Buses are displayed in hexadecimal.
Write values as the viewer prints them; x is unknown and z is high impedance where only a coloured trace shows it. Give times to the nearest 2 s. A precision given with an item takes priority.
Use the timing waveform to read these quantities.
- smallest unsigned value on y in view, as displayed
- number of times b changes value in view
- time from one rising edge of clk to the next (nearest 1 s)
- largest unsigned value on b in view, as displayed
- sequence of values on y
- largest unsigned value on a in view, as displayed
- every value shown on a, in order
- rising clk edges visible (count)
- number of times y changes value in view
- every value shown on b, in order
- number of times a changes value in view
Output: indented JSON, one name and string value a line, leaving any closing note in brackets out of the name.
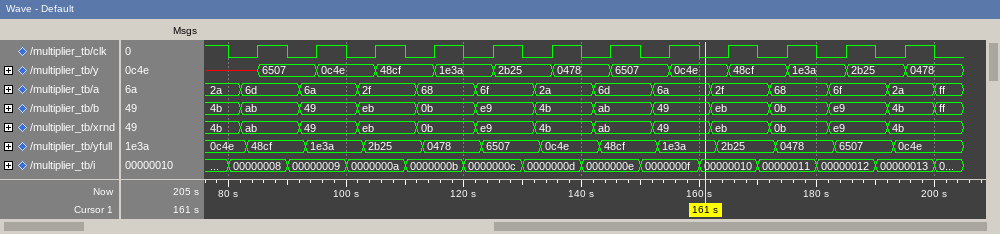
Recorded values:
{
  "smallest unsigned value on y in view, as displayed": "0478",
  "number of times b changes value in view": "13",
  "time from one rising edge of clk to the next": "10 s",
  "largest unsigned value on b in view, as displayed": "ff",
  "sequence of values on y": "x, 6507, 0c4e, 48cf, 1e3a, 2b25, 0478, 6507, 0c4e, 48cf, 1e3a, 2b25, 0478",
  "largest unsigned value on a in view, as displayed": "ff",
  "every value shown on a, in order": "2a, 6d, 6a, 2f, 68, 6f, 2a, 6d, 6a, 2f, 68, 6f, 2a, ff",
  "rising clk edges visible": "12",
  "number of times y changes value in view": "12",
  "every value shown on b, in order": "4b, ab, 49, eb, 0b, e9, 4b, ab, 49, eb, 0b, e9, 4b, ff",
  "number of times a changes value in view": "13"
}
